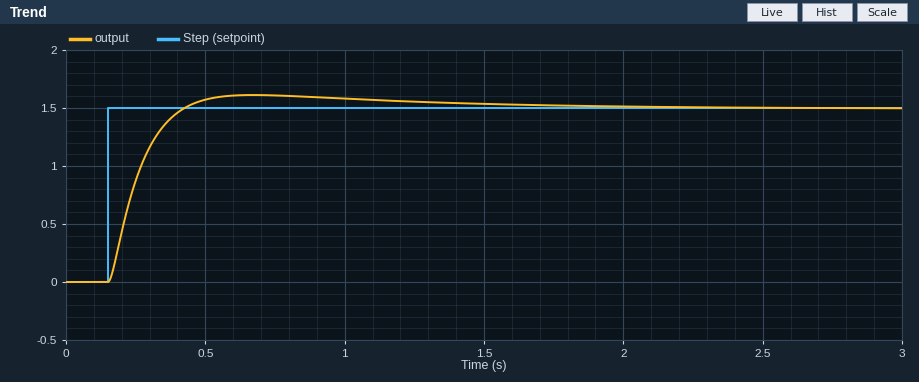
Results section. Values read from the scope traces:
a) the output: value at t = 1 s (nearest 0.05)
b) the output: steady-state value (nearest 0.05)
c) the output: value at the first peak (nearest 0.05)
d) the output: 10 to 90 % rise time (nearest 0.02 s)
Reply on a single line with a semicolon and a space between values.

1.60; 1.50; 1.60; 0.18 s
